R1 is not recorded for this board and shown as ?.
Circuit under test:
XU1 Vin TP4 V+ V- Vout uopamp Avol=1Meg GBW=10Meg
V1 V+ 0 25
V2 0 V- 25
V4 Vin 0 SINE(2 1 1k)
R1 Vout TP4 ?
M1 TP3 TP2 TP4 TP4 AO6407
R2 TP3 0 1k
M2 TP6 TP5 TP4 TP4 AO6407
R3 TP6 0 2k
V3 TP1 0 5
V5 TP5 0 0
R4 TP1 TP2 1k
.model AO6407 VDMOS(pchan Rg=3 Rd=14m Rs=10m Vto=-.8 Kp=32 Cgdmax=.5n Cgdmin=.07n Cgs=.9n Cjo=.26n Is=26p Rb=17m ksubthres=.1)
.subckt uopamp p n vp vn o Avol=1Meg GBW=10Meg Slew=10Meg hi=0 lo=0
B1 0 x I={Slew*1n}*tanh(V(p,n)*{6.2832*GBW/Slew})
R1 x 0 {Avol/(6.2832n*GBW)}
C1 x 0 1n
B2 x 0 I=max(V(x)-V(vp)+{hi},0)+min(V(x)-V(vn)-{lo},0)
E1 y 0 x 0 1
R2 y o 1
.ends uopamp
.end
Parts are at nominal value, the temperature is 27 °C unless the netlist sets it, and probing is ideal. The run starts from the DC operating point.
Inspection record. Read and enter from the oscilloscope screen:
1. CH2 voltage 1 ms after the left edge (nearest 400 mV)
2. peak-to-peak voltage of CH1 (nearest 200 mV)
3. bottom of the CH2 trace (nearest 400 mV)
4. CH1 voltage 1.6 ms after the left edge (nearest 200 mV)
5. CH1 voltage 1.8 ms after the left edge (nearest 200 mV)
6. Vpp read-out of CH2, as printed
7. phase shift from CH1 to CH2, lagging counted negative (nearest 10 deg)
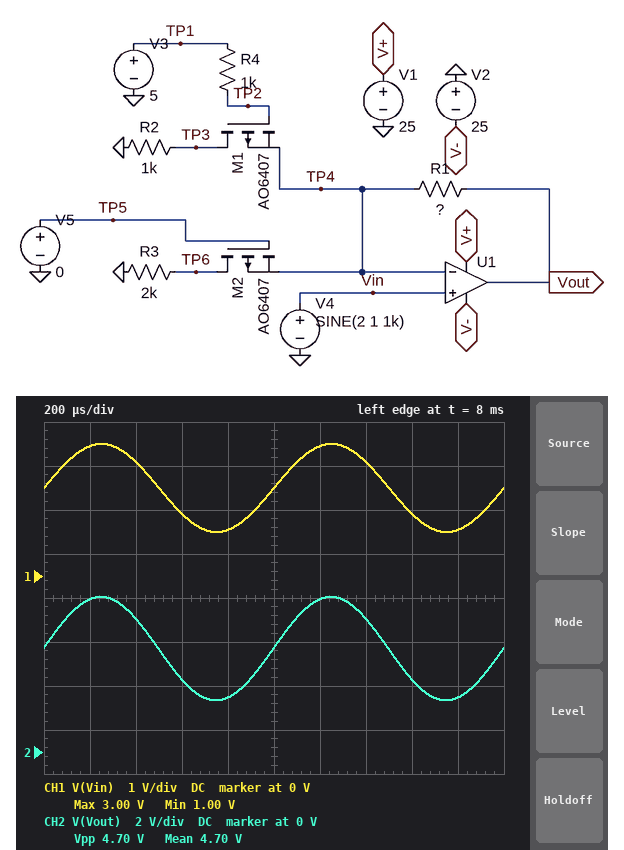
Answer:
4.8 V
2.0 V
2.4 V
1.4 V
1.0 V
4.70 V
0 deg
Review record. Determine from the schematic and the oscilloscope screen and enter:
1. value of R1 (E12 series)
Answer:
2.7 kΩ
